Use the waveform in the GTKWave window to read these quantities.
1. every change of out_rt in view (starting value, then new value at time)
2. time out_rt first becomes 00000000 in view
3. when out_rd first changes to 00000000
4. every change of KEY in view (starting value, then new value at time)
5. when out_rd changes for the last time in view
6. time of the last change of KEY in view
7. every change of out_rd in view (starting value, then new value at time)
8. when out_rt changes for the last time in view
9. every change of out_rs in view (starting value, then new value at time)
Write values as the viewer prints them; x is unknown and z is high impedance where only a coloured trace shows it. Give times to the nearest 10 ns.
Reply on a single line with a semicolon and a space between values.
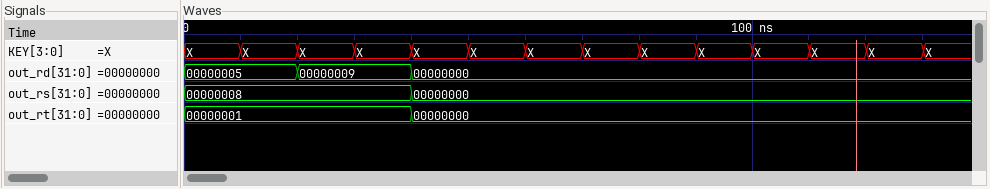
00000001, 00000000 at 40 ns; 40 ns; 40 ns; X, X at 10 ns, X at 20 ns, X at 30 ns, X at 40 ns, X at 50 ns, X at 60 ns, X at 70 ns, X at 80 ns, X at 90 ns, X at 100 ns, X at 110 ns, X at 120 ns, X at 130 ns; 40 ns; 130 ns; 00000005, 00000009 at 20 ns, 00000000 at 40 ns; 40 ns; 00000008, 00000000 at 40 ns
